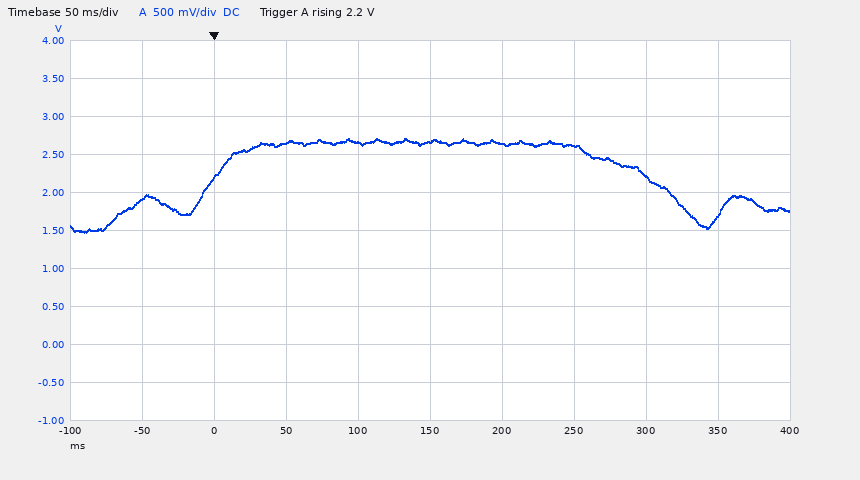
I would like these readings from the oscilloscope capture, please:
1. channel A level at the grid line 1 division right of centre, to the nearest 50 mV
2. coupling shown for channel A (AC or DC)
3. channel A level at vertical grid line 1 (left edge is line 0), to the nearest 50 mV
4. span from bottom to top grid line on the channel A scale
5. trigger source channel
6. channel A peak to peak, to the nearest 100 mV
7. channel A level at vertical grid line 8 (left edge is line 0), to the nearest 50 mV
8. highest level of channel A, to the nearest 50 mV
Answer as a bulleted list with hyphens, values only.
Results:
- 2.65 V
- DC
- 1.90 V
- 5 V
- channel A
- 1.20 V
- 2.20 V
- 2.70 V
